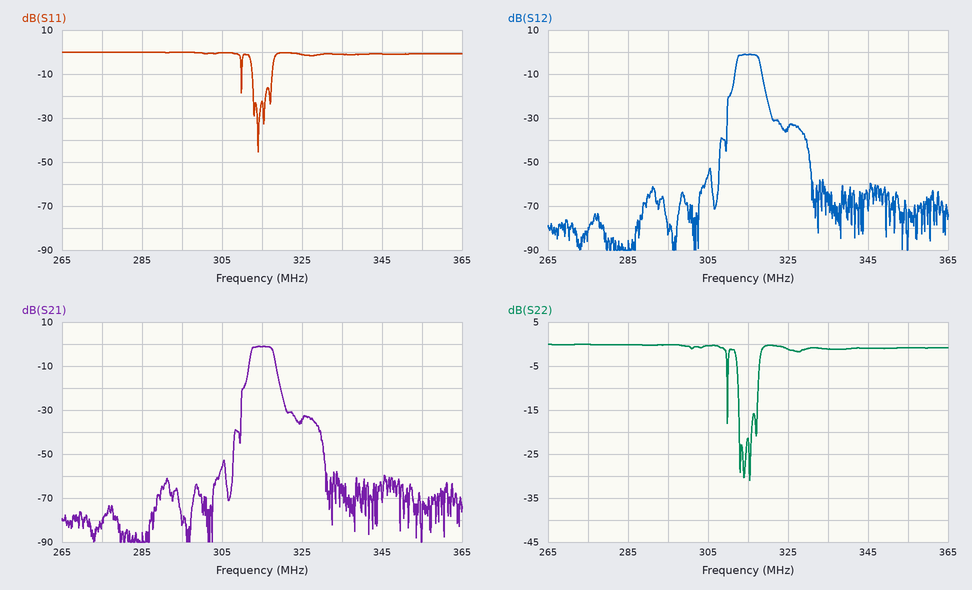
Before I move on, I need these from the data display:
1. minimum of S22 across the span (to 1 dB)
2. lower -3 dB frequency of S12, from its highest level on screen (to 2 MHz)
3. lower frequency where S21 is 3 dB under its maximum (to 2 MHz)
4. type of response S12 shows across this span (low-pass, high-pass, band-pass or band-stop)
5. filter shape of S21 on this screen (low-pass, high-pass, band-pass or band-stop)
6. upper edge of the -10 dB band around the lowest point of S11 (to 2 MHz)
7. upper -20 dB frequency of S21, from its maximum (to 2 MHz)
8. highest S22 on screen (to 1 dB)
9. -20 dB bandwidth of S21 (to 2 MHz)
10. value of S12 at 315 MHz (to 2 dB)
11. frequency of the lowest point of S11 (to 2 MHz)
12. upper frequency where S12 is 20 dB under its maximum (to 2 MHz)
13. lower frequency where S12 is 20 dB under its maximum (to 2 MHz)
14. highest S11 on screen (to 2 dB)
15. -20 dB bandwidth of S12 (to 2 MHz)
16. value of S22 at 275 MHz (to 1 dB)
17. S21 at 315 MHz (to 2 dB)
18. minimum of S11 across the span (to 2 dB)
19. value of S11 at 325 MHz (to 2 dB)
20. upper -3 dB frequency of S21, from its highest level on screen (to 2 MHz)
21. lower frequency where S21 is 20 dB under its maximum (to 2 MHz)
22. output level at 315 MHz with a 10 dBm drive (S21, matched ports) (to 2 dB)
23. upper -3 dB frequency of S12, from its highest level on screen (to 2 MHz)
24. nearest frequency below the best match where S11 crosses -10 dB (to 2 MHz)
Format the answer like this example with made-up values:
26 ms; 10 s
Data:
-31 dB; 312 MHz; 312 MHz; band-pass; band-pass; 318 MHz; 320 MHz; 0 dB; 10 MHz; -2 dB; 314 MHz; 320 MHz; 310 MHz; 0 dB; 10 MHz; 0 dB; -2 dB; -46 dB; -2 dB; 318 MHz; 310 MHz; 8 dBm; 318 MHz; 312 MHz
